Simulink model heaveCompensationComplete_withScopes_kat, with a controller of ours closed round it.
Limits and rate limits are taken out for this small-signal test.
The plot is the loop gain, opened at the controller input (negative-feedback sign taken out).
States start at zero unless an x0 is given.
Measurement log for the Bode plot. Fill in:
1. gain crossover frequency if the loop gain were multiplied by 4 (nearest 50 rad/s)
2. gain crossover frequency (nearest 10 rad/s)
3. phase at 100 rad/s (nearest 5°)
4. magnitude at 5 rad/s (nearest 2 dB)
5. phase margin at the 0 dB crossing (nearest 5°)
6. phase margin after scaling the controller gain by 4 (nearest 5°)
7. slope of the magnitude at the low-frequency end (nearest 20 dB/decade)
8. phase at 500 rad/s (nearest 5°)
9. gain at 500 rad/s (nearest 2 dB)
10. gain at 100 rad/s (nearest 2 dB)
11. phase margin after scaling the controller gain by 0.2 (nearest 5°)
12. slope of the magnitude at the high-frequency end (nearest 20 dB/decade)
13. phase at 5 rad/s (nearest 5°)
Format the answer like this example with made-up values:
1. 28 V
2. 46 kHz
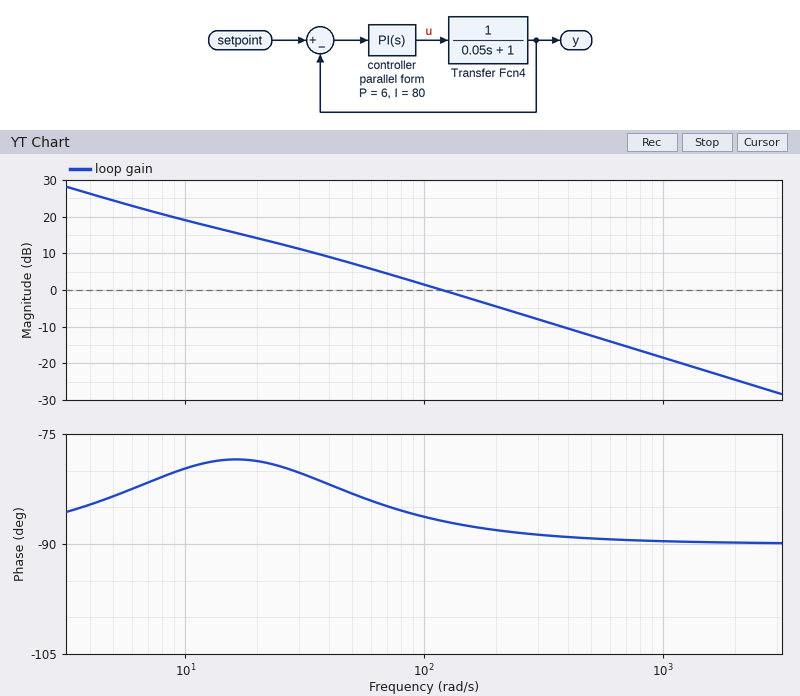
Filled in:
1. 500 rad/s
2. 120 rad/s
3. -85°
4. 24 dB
5. 95°
6. 90°
7. -20 dB/decade
8. -90°
9. -12 dB
10. 2 dB
11. 100°
12. -20 dB/decade
13. -85°
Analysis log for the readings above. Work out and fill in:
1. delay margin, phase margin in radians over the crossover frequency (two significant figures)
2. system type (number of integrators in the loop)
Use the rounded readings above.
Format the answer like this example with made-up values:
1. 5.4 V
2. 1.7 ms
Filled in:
1. 0.014 s
2. 1
